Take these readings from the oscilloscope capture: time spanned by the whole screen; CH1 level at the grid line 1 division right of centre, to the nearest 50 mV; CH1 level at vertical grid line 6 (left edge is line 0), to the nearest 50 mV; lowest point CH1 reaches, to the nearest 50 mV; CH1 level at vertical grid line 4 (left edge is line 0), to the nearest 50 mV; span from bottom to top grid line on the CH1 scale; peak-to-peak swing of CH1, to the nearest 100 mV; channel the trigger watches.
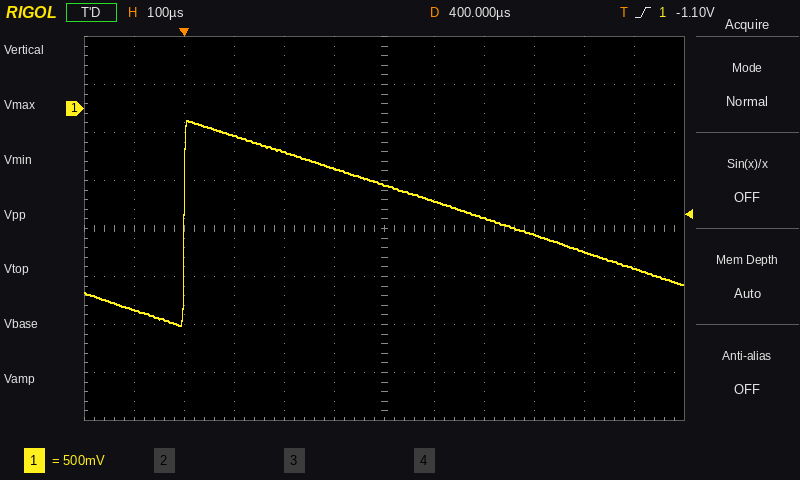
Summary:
1.2 ms
-950 mV
-800 mV
-2.25 V
-450 mV
4 V
2.10 V
CH1
